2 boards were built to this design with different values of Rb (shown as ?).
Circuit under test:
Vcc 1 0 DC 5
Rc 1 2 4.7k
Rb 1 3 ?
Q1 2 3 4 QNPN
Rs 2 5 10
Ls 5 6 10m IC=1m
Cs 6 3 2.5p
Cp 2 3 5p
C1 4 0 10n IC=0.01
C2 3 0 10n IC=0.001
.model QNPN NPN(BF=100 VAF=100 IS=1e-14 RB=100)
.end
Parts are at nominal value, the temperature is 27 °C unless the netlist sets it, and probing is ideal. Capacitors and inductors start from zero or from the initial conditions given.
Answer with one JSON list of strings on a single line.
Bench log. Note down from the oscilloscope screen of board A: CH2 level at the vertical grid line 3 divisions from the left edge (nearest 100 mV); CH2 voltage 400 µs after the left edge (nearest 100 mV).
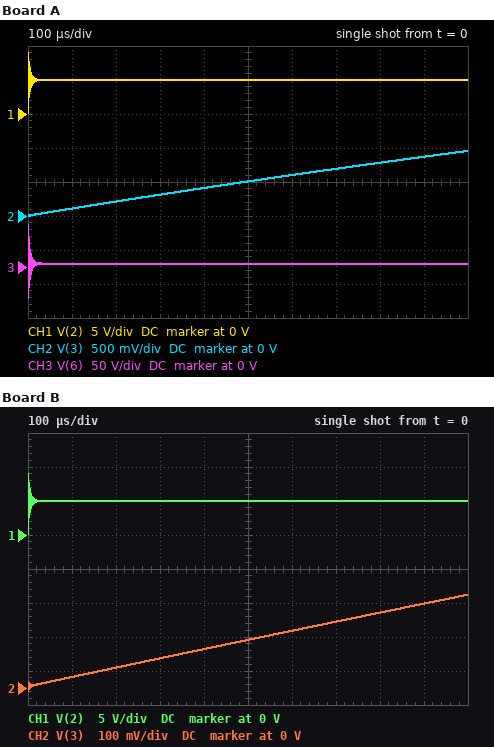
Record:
["300 mV", "400 mV"]
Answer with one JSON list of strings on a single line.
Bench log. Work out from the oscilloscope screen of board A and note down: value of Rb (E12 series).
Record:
["470 kΩ"]
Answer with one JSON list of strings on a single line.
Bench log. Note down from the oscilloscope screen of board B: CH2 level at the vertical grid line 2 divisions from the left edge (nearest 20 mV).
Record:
["60 mV"]
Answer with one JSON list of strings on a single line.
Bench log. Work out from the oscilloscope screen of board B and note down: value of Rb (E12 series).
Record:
["1.8 MΩ"]
